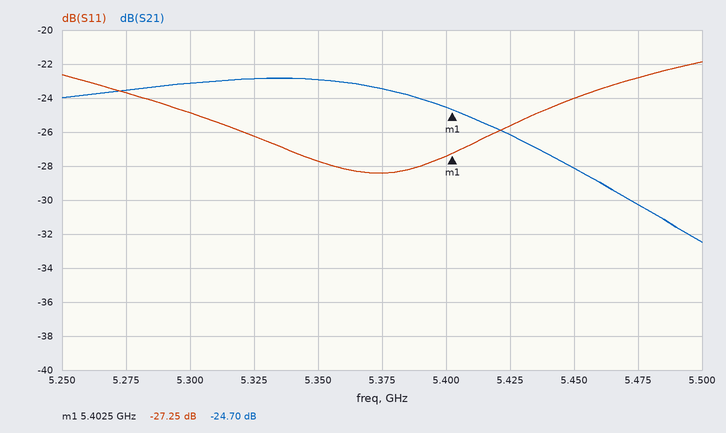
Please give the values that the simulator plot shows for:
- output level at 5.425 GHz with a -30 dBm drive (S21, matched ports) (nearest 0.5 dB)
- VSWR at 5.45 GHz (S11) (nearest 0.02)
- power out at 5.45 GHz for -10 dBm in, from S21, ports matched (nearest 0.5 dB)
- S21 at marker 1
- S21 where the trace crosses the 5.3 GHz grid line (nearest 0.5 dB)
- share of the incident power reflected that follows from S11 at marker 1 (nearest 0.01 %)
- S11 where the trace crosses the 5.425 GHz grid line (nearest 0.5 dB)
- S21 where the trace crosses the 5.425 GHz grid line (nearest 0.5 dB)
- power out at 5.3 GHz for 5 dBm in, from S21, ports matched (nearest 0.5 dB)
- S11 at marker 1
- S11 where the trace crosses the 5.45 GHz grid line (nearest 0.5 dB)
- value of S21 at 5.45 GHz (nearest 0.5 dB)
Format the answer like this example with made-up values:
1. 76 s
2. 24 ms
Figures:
1. -56.0 dBm
2. 1.14
3. -38.0 dBm
4. -24.70 dB
5. -23.0 dB
6. 0.19 %
7. -25.5 dB
8. -26.0 dB
9. -18.0 dBm
10. -27.25 dB
11. -24.0 dB
12. -28.0 dB
